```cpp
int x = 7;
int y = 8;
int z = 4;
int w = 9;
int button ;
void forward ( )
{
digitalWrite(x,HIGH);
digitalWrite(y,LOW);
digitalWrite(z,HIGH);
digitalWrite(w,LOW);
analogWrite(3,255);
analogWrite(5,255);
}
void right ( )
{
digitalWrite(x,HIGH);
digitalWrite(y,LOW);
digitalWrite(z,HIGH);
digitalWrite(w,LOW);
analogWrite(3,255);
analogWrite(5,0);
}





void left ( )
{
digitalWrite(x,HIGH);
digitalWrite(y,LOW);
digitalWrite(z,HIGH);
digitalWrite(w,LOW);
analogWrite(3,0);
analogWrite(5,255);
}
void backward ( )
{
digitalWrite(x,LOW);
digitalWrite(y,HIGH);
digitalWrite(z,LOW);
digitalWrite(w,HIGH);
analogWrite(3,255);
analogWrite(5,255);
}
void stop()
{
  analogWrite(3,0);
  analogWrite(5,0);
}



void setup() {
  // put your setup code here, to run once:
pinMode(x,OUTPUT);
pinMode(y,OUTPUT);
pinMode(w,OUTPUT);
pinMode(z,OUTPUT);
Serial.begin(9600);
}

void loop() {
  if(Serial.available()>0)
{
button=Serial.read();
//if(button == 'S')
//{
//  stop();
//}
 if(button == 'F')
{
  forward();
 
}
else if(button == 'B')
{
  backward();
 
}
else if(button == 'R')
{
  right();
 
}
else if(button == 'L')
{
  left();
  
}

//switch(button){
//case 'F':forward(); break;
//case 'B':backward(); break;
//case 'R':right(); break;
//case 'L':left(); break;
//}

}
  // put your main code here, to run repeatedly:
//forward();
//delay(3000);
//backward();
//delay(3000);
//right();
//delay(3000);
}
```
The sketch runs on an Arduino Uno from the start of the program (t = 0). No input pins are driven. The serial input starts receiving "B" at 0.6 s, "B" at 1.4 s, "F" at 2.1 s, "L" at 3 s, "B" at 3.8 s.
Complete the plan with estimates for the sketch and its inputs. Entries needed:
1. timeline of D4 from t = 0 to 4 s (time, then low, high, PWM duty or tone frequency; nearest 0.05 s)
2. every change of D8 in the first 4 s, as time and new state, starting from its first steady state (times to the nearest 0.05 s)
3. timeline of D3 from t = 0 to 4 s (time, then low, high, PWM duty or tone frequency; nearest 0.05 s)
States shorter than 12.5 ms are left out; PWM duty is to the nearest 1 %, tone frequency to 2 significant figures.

0 s low; 2.1 s high; 3.8 s low
0 s low; 0.6 s high; 2.1 s low; 3.8 s high
0.6 s high; 3 s low; 3.8 s high
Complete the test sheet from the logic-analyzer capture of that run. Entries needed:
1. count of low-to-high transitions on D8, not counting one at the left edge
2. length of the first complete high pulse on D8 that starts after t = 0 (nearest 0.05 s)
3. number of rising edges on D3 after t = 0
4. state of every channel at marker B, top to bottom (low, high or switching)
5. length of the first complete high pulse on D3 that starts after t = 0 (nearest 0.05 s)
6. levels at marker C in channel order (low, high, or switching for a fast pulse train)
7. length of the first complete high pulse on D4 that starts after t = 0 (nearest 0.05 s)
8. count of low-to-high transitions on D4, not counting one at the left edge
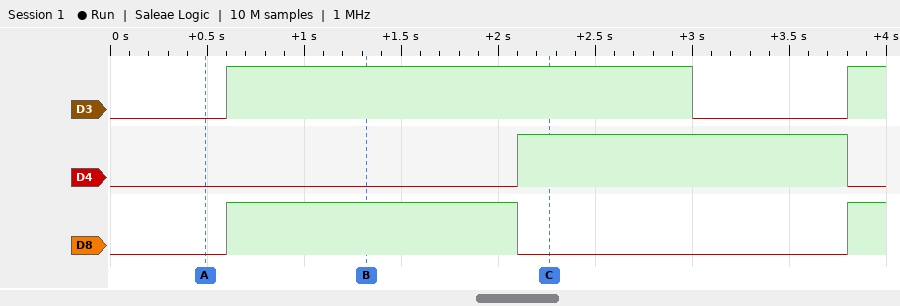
2
1.50 s
2
D3 high, D4 low, D8 high
2.40 s
D3 high, D4 high, D8 low
1.70 s
1
